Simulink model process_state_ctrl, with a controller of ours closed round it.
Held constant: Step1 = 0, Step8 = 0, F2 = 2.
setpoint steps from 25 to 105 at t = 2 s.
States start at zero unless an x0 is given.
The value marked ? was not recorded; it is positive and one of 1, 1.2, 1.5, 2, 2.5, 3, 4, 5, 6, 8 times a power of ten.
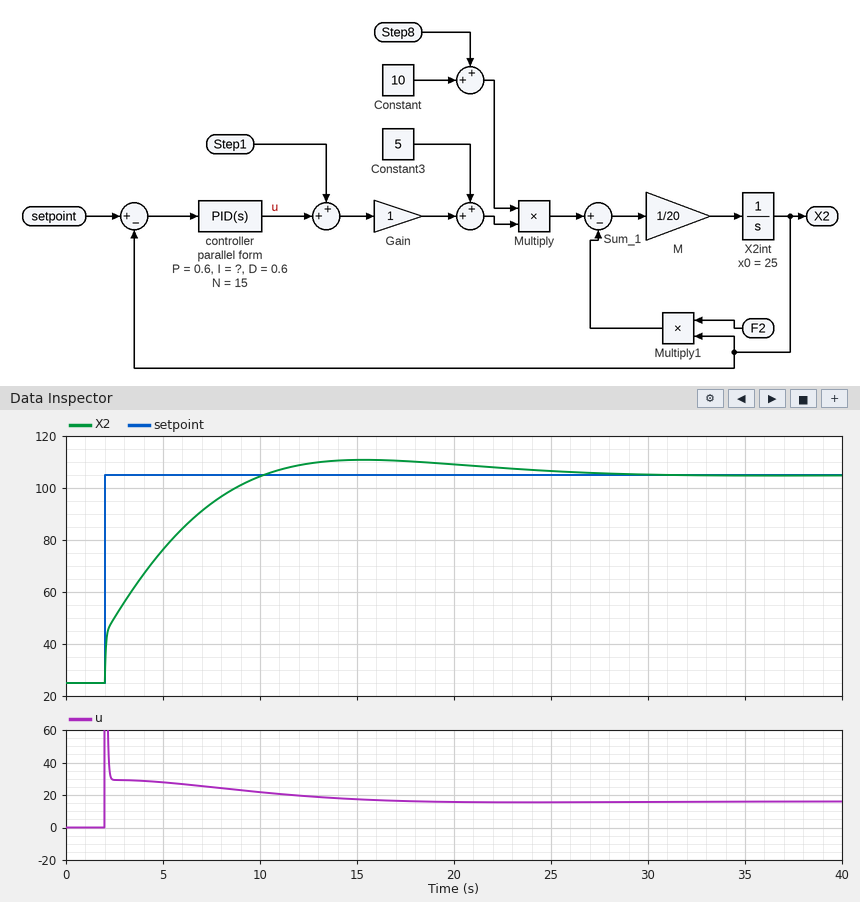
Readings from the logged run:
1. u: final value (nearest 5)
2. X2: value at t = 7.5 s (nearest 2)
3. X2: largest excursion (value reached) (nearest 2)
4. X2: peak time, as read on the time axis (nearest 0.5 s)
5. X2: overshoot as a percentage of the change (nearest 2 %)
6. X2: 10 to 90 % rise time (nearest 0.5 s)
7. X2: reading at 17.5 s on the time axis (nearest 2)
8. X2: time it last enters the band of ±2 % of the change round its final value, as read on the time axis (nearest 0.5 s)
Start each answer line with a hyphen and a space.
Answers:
- 15
- 94
- 110
- 15.5 s
- 8 %
- 6.0 s
- 110
- 25.0 s
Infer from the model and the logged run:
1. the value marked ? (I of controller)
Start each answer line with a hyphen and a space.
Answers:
- 0.12
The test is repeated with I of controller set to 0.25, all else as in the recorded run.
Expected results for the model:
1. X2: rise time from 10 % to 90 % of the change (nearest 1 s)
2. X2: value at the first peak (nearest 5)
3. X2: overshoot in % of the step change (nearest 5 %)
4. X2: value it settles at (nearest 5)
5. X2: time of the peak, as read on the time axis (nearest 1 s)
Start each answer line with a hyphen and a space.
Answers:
- 4 s
- 120
- 15 %
- 105
- 11 s
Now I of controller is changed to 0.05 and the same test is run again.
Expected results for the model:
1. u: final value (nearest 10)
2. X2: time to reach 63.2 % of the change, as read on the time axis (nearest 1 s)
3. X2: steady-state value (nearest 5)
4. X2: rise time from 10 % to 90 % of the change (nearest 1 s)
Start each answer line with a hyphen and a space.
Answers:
- 20
- 6 s
- 105
- 10 s
